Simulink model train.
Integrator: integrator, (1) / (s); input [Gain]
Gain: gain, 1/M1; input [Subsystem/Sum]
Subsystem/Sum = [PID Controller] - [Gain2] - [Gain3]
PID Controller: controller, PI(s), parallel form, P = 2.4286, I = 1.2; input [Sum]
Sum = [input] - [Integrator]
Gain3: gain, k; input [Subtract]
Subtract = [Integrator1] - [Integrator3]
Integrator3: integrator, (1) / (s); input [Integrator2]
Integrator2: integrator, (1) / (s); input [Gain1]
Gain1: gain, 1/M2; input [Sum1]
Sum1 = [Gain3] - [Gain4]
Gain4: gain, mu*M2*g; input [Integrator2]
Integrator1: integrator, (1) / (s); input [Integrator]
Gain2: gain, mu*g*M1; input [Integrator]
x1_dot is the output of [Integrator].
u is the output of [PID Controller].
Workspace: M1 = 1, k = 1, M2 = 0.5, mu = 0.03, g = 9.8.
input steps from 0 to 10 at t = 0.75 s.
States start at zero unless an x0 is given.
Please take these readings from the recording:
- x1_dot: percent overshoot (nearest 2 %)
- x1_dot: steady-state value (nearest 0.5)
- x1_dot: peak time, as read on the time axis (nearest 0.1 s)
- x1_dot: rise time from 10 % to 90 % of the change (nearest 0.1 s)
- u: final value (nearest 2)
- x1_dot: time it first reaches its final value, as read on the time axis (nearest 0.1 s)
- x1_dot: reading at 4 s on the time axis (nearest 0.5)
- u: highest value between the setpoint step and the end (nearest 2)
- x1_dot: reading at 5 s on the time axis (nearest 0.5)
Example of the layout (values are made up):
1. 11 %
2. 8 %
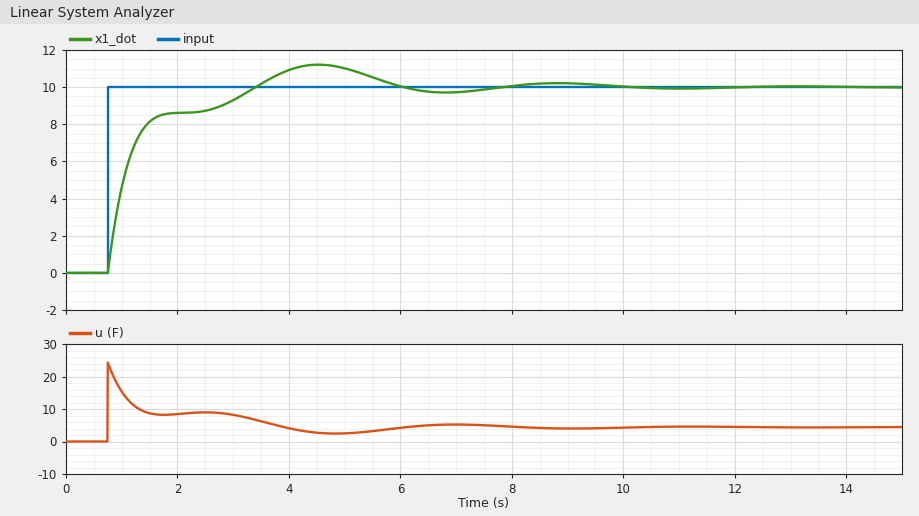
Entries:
1. 12 %
2. 10.0
3. 4.5 s
4. 2.0 s
5. 4
6. 3.4 s
7. 11.0
8. 24
9. 11.0
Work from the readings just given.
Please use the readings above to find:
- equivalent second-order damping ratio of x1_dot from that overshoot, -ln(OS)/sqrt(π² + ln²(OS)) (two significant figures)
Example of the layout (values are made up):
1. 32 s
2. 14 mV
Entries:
1. 0.56
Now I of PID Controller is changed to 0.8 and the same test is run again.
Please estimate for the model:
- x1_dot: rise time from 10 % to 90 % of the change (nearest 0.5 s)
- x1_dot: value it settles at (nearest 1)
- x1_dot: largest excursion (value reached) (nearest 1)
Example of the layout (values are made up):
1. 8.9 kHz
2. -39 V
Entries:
1. 2.5 s
2. 10
3. 11
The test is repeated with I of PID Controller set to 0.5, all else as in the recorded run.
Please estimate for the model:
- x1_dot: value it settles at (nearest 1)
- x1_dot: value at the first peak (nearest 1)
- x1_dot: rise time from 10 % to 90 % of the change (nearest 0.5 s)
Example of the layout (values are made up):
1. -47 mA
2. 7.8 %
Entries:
1. 10
2. 10
3. 2.5 s
